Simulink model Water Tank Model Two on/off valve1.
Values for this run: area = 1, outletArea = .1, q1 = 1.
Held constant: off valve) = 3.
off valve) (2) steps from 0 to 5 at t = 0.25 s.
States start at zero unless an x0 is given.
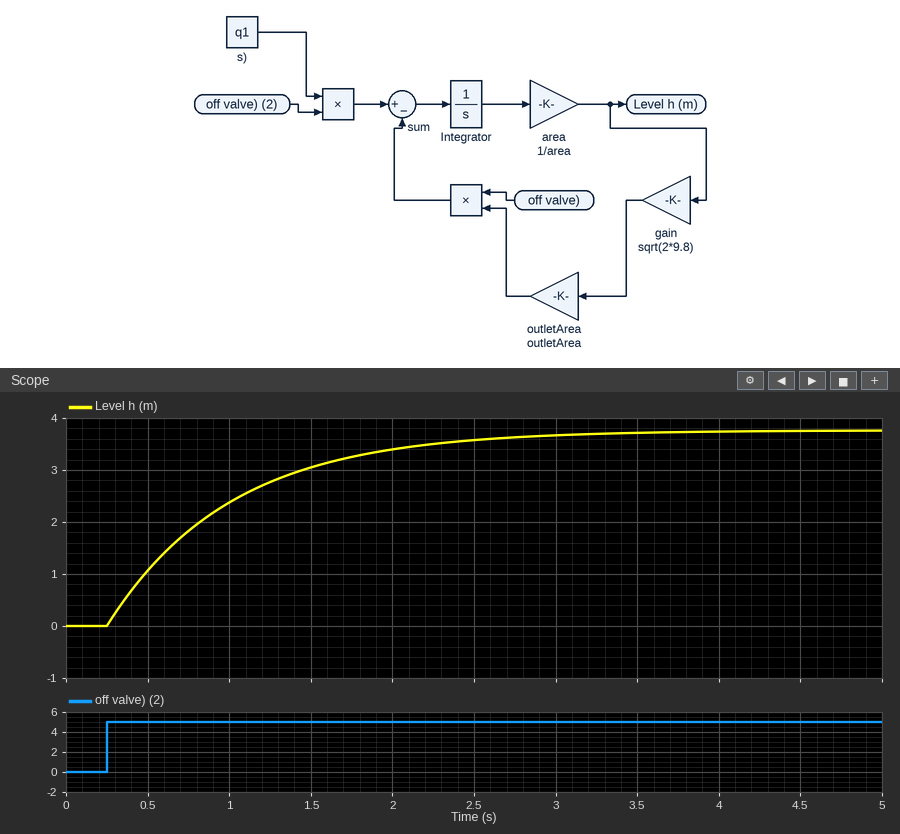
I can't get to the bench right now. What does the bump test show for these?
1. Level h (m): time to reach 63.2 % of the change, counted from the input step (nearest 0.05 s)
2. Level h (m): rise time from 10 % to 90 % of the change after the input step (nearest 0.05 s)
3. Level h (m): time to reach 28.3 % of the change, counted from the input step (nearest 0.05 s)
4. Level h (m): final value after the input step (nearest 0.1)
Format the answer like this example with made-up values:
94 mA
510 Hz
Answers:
0.75 s
1.65 s
0.25 s
3.8
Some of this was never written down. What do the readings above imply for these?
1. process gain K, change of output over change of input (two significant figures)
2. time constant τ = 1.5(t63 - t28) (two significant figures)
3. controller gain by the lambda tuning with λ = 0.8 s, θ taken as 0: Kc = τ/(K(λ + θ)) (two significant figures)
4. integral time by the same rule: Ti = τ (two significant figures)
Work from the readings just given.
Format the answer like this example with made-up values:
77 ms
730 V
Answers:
0.76
0.75 s
1.2
0.75 s
